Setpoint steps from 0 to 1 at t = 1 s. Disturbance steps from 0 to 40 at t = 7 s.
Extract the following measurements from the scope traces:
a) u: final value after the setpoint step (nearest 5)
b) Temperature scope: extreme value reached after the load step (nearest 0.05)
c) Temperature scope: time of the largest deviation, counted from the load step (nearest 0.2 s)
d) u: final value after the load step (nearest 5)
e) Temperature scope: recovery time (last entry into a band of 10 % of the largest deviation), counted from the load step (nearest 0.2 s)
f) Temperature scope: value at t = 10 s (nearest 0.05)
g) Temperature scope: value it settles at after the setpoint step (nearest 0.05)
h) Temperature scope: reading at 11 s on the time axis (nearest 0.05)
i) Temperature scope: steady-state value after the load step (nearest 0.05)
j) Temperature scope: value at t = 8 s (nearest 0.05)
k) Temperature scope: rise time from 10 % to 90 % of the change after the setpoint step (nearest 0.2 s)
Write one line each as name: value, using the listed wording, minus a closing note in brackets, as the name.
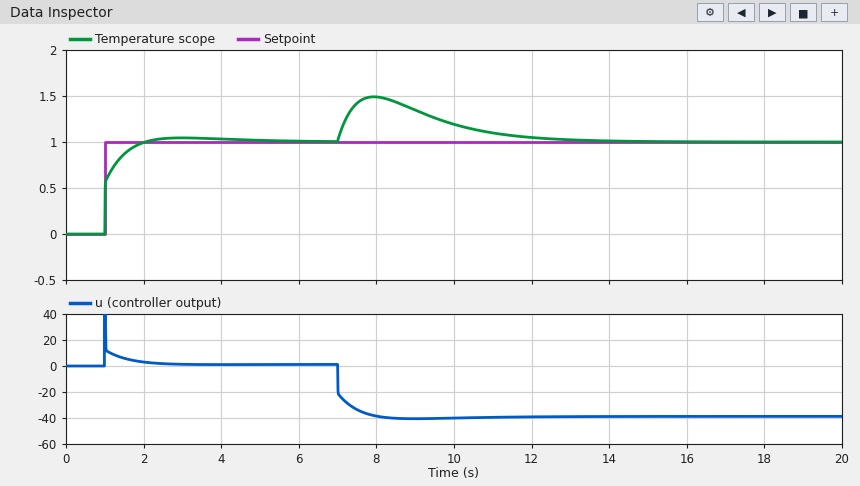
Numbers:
u: final value after the setpoint step: 0
Temperature scope: extreme value reached after the load step: 1.50
Temperature scope: time of the largest deviation, counted from the load step: 1.0 s
u: final value after the load step: -40
Temperature scope: recovery time (last entry into a band of 10 % of the largest deviation), counted from the load step: 5.0 s
Temperature scope: value at t = 10 s: 1.20
Temperature scope: value it settles at after the setpoint step: 1.00
Temperature scope: reading at 11 s on the time axis: 1.10
Temperature scope: steady-state value after the load step: 1.00
Temperature scope: value at t = 8 s: 1.50
Temperature scope: rise time from 10 % to 90 % of the change after the setpoint step: 0.6 s
